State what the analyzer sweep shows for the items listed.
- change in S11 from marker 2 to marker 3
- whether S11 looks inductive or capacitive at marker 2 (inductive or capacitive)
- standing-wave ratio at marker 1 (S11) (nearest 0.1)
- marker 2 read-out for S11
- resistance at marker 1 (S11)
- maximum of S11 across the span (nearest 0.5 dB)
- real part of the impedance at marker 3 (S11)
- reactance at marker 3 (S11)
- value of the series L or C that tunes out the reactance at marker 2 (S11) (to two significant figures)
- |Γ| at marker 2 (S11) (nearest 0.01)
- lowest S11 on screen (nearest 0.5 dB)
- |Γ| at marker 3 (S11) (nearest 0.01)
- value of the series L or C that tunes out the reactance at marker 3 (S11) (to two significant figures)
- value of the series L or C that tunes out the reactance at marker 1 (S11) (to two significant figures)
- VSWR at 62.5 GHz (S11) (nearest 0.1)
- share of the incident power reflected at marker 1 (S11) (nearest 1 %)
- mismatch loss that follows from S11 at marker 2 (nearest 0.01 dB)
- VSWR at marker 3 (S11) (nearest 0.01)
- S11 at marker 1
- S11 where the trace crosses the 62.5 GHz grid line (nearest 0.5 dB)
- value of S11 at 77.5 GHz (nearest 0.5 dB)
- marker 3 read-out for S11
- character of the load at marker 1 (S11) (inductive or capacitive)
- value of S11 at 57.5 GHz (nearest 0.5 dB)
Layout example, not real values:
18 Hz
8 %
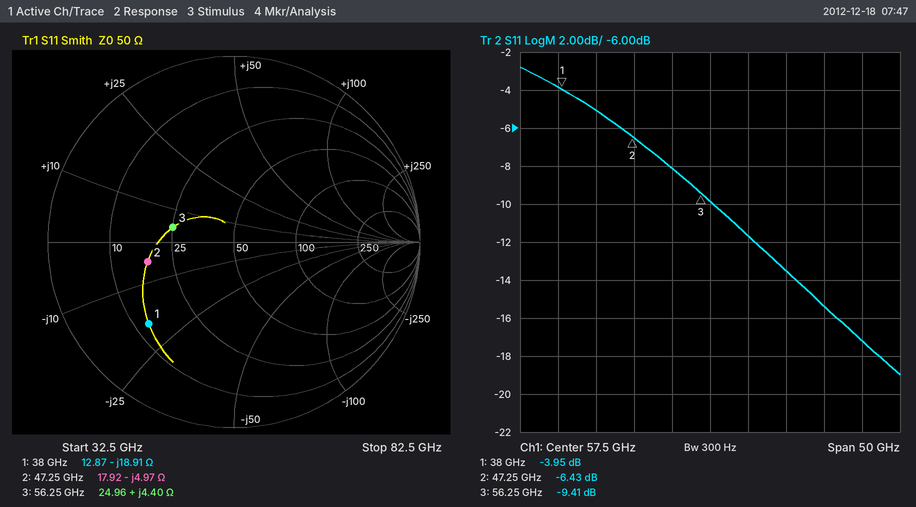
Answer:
-2.98 dB
capacitive
4.5
-6.43 dB
12.87 Ω
-3.0 dB
24.96 Ω
+4.40 Ω
17 pH
0.48
-19.0 dB
0.34
640 fF
79 pH
1.7
40 %
1.12 dB
2.02
-3.95 dB
-11.5 dB
-17.0 dB
-9.41 dB
capacitive
-10.0 dB
